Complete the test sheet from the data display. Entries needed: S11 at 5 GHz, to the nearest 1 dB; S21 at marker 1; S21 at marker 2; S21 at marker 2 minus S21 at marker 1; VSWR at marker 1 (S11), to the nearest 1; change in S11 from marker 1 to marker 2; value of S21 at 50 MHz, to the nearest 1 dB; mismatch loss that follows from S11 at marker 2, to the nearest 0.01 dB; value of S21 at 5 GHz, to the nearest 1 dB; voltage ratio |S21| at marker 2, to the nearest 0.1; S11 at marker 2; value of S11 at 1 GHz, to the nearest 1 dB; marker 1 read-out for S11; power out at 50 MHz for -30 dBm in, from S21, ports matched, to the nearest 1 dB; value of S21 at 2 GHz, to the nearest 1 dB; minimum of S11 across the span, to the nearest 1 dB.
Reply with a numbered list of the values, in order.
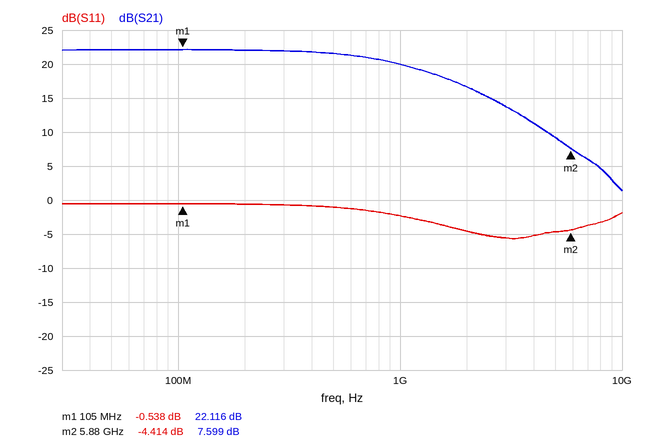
1. -5 dB
2. 22.116 dB
3. 7.599 dB
4. -14.517 dB
5. 32
6. -3.876 dB
7. 22 dB
8. 1.95 dB
9. 9 dB
10. 2.4
11. -4.414 dB
12. -2 dB
13. -0.538 dB
14. -8 dBm
15. 17 dB
16. -6 dB
